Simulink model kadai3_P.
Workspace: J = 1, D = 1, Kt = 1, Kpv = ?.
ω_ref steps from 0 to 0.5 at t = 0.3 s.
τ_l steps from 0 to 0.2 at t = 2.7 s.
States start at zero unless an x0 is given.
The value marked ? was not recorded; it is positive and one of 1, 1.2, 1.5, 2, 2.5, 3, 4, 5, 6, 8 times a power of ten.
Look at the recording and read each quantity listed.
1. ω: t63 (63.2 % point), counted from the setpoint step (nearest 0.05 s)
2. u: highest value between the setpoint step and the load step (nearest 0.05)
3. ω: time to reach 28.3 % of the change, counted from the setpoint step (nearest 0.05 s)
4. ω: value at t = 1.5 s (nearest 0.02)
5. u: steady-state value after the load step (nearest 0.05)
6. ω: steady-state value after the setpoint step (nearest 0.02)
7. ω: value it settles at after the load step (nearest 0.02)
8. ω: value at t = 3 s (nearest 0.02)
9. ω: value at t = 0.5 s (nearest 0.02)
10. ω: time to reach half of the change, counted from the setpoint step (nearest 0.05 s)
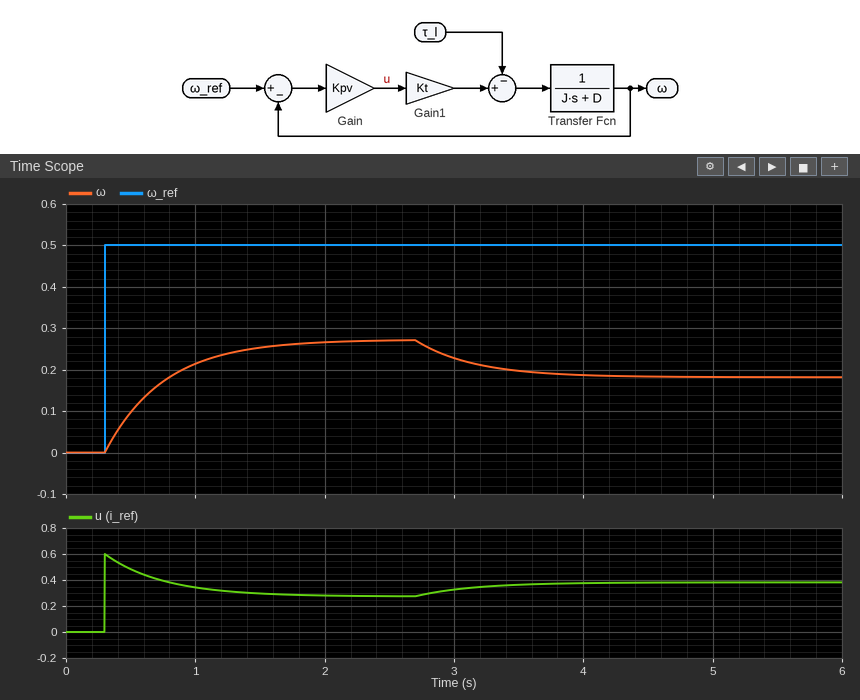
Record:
0.45 s
0.60
0.15 s
0.26
0.40
0.28
0.18
0.22
0.10
0.30 s
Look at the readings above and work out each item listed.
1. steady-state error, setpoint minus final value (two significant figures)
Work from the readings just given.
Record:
0.22
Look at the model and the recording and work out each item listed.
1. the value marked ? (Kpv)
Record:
1.2
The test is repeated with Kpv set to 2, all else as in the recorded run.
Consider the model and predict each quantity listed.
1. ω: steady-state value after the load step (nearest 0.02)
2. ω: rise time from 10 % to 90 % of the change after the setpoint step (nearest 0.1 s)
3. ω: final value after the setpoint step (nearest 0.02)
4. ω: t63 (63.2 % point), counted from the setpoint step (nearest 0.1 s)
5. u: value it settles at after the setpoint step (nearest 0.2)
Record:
0.26
0.7 s
0.34
0.3 s
0.4
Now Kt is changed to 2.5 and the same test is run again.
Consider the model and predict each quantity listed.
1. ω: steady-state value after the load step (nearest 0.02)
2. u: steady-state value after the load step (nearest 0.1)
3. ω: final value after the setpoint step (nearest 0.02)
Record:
0.32
0.2
0.38
